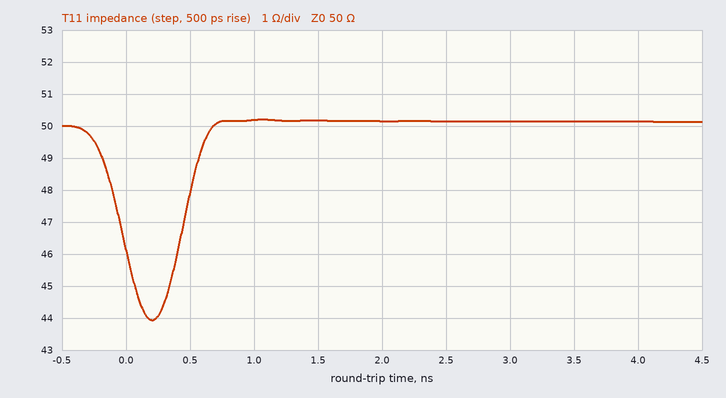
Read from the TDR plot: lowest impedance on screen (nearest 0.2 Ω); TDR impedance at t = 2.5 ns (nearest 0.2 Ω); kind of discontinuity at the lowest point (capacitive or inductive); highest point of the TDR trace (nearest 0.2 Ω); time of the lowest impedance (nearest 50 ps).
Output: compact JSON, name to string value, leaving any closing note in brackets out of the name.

{"lowest impedance on screen": "44.0 Ω", "TDR impedance at t = 2.5 ns": "50.2 Ω", "kind of discontinuity at the lowest point": "capacitive", "highest point of the TDR trace": "50.2 Ω", "time of the lowest impedance": "200 ps"}
